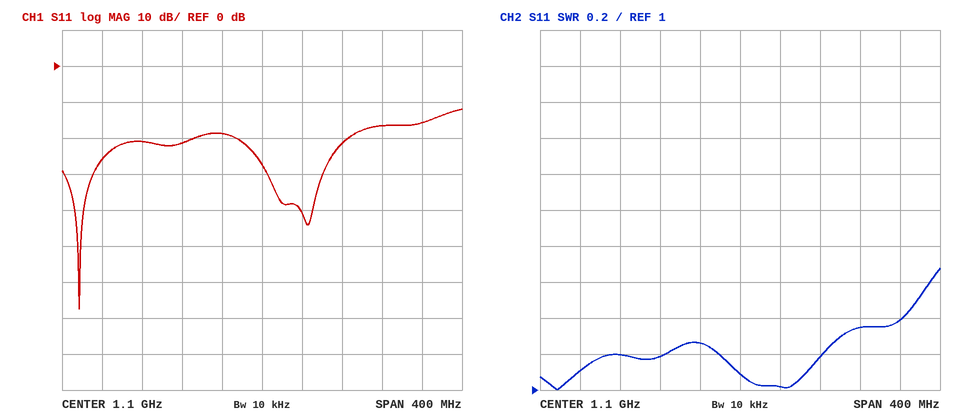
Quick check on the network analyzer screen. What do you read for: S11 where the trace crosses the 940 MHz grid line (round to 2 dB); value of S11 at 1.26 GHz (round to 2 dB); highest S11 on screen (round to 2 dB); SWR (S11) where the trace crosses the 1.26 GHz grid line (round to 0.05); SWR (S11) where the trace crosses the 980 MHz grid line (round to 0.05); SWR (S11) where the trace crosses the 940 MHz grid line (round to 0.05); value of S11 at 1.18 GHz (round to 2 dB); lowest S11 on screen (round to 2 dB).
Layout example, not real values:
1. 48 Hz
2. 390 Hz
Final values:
1. -26 dB
2. -16 dB
3. -12 dB
4. 1.40
5. 1.20
6. 1.10
7. -22 dB
8. -68 dB
